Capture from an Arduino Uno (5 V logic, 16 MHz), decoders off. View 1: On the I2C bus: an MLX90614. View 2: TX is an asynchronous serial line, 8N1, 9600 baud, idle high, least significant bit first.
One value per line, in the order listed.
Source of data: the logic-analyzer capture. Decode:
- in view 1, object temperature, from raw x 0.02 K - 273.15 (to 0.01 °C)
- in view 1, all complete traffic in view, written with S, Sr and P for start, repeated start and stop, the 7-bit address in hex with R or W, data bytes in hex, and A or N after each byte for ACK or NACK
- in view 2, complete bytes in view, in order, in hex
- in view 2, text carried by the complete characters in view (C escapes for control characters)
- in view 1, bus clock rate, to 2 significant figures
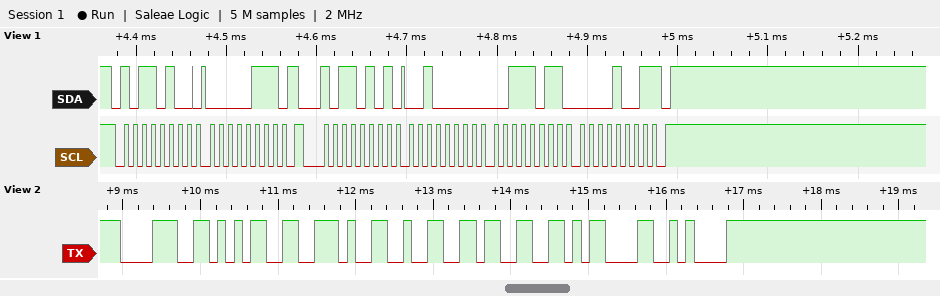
29.57 °C
S 5AW A 07 A Sr 5AR A 20 A 3B A 09 N P
38 35 2E 32 33 0D 0A
"85.23\r\n"
100 kHz
